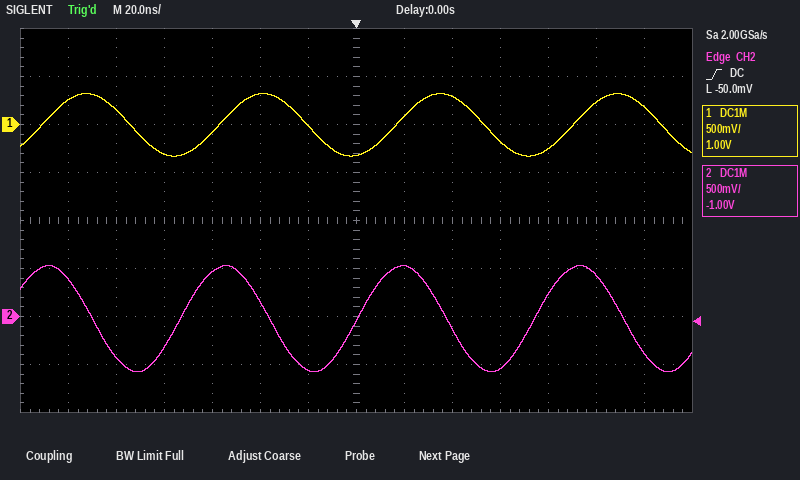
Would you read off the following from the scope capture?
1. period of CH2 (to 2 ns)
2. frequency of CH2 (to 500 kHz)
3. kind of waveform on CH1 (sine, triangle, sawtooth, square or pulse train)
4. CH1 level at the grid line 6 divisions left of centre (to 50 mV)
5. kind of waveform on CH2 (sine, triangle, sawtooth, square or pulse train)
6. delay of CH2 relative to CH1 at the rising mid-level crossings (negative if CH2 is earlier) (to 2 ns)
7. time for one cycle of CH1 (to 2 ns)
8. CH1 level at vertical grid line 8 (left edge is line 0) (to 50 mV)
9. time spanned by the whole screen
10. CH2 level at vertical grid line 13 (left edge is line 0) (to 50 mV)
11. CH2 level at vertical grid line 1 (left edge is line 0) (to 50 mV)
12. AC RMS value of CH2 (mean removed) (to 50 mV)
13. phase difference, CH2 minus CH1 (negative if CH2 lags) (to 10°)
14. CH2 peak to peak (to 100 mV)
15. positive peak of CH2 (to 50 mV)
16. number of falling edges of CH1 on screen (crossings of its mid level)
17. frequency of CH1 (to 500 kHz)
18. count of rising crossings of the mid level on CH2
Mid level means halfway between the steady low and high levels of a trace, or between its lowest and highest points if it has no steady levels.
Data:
74 ns
13.5 MHz
sine
250 mV
sine
-16 ns
74 ns
100 mV
280 ns
-400 mV
400 mV
400 mV
+80°
1.10 V
550 mV
4
13.5 MHz
3
